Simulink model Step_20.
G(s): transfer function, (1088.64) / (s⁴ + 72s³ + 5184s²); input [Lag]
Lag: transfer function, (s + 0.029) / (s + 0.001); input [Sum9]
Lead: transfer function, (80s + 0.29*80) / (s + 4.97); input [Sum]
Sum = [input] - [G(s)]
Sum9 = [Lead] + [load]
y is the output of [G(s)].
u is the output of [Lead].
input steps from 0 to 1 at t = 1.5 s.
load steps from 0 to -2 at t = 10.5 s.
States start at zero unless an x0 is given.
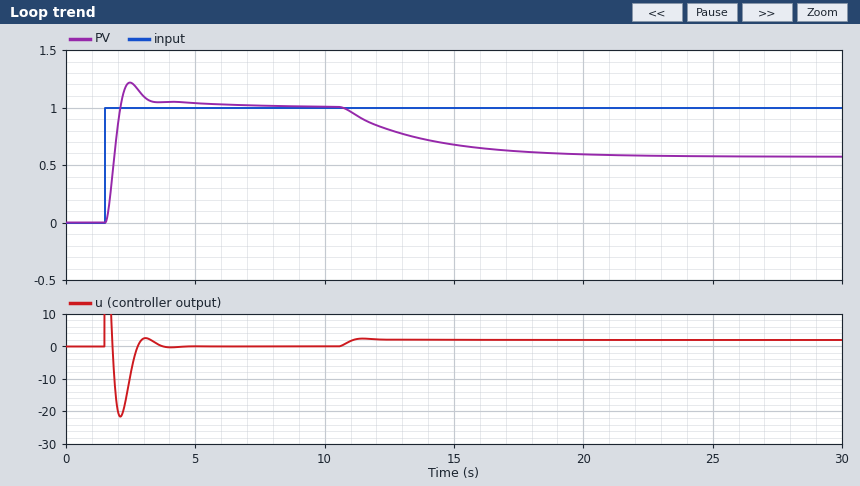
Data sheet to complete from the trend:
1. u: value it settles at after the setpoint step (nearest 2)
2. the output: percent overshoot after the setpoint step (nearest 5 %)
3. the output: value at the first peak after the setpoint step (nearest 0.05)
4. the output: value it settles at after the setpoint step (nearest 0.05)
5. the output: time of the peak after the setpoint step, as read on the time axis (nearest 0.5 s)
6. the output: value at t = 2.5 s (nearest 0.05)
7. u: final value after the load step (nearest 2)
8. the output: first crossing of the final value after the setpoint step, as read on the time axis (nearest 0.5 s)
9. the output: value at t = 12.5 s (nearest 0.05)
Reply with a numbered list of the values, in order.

1. 0
2. 20 %
3. 1.20
4. 1.00
5. 2.5 s
6. 1.20
7. 2
8. 2.0 s
9. 0.80
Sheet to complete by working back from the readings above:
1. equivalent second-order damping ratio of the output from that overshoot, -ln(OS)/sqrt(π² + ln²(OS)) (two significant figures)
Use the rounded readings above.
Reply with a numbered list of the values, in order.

1. 0.46
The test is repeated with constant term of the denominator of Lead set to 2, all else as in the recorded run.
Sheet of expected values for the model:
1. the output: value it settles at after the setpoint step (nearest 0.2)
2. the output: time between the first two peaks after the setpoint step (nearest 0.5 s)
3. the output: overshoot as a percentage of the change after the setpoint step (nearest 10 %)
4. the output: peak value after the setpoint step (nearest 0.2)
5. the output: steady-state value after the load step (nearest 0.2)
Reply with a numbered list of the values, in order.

1. 1.0
2. 1.5 s
3. 60 %
4. 1.6
5. 0.8
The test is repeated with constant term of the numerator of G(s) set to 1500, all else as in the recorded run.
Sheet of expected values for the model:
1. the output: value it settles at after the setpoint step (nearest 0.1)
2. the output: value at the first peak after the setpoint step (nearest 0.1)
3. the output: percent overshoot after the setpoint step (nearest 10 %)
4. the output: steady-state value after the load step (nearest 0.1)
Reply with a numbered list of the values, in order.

1. 1.0
2. 1.3
3. 30 %
4. 0.6
